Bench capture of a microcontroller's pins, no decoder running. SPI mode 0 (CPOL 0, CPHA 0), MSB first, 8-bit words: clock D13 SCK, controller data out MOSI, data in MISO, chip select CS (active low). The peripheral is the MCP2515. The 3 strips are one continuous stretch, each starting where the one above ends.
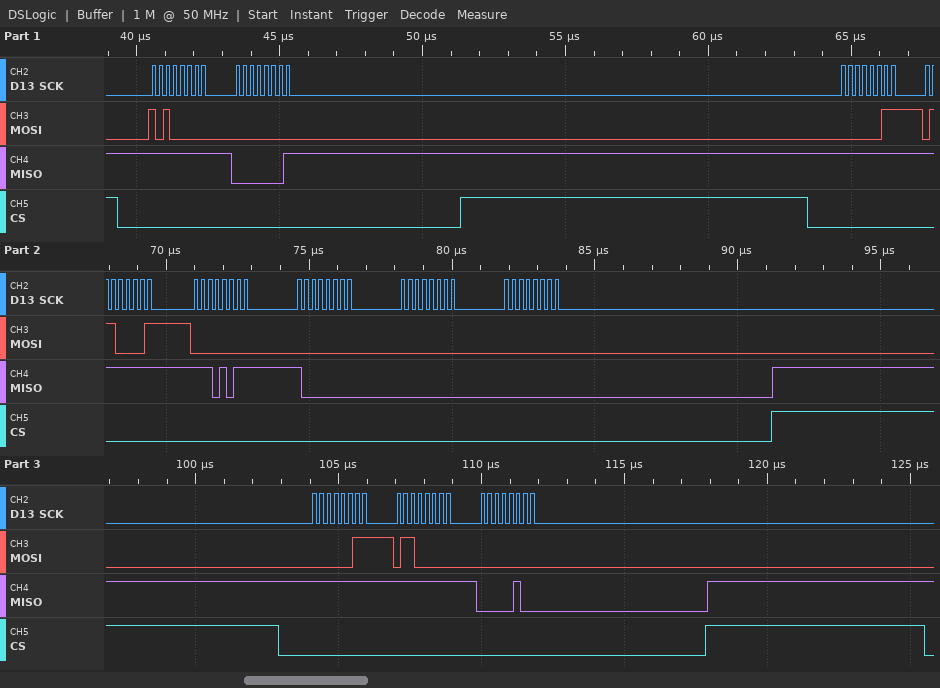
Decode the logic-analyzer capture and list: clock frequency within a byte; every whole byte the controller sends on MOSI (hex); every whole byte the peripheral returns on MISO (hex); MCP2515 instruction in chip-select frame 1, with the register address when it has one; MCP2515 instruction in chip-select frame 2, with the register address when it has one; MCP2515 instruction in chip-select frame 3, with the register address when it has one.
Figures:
4 MHz
A0 00 03 61 00 00 00 00 03 60 00
FF 01 FF FF EB 80 00 00 FF FF 04
READ STATUS
READ 0x61
READ 0x60
